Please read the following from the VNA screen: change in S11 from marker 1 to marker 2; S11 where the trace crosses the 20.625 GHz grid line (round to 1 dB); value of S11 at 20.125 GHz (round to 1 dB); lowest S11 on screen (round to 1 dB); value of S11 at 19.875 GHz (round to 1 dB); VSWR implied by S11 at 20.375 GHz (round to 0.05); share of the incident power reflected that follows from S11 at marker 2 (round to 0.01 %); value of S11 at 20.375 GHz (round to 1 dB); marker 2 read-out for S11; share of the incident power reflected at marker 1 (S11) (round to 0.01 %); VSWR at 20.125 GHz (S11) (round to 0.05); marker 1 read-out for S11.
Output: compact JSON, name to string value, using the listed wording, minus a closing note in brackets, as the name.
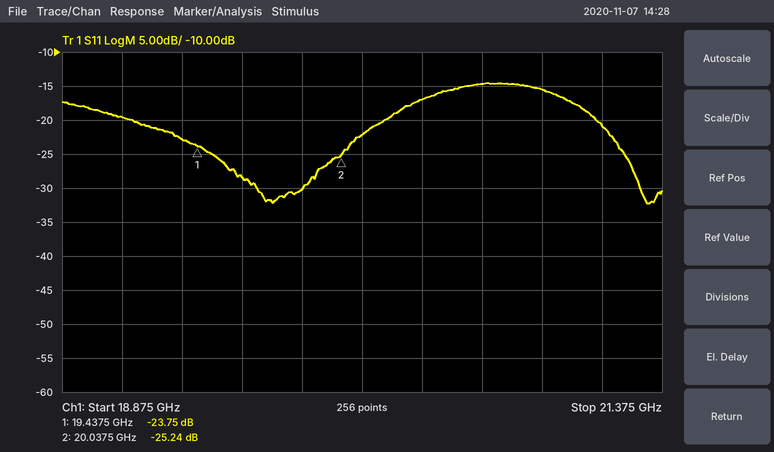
{"change in S11 from marker 1 to marker 2": "-1.49 dB", "S11 where the trace crosses the 20.625 GHz grid line": "-15 dB", "value of S11 at 20.125 GHz": "-22 dB", "lowest S11 on screen": "-32 dB", "value of S11 at 19.875 GHz": "-30 dB", "VSWR implied by S11 at 20.375 GHz": "1.35", "share of the incident power reflected that follows from S11 at marker 2": "0.30 %", "value of S11 at 20.375 GHz": "-17 dB", "marker 2 read-out for S11": "-25.24 dB", "share of the incident power reflected at marker 1 (S11)": "0.42 %", "VSWR at 20.125 GHz (S11)": "1.15", "marker 1 read-out for S11": "-23.75 dB"}
